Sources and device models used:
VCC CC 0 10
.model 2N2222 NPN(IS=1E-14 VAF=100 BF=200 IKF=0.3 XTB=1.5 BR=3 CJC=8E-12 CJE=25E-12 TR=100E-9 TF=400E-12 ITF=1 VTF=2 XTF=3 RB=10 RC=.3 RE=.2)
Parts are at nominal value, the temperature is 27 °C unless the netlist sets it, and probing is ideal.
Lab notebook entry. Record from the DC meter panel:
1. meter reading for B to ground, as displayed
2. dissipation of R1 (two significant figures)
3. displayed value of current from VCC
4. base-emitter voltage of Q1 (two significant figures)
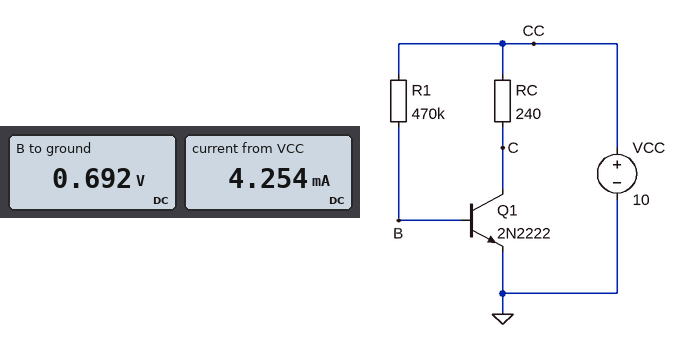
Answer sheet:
0.692 V
180 µW
4.254 mA
690 mV
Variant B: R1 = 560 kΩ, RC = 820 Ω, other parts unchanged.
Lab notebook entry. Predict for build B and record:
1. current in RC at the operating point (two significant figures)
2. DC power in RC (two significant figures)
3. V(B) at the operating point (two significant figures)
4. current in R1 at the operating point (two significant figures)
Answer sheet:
3.5 mA
10 mW
690 mV
17 µA
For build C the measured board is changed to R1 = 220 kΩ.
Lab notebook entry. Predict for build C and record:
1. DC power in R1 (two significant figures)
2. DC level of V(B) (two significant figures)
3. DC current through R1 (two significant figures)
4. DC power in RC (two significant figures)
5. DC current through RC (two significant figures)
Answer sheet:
390 µW
710 mV
42 µA
19 mW
8.8 mA
